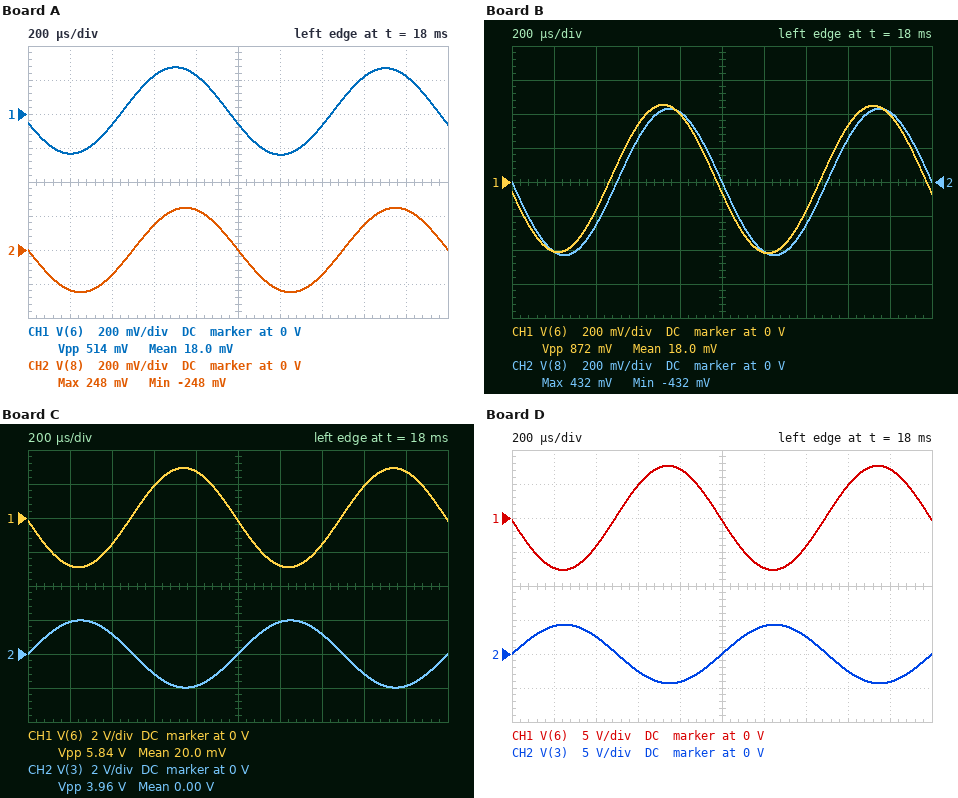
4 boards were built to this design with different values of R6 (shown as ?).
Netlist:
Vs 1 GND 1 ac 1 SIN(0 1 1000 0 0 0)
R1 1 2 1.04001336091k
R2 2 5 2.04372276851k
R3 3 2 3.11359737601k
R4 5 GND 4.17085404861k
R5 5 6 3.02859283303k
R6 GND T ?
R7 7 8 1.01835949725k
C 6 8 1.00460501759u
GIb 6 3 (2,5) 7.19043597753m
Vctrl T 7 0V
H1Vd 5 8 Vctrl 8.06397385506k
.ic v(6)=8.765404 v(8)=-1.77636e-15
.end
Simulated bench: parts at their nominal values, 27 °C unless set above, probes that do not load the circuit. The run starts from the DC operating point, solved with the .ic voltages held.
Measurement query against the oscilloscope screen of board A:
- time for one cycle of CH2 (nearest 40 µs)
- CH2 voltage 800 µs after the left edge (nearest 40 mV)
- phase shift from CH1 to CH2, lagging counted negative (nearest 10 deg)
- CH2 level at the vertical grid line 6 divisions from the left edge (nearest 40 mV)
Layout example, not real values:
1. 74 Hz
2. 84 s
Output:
1. 1.00 ms
2. 240 mV
3. -20 deg
4. -240 mV
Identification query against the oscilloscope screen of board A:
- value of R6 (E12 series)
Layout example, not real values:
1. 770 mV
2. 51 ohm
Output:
1. 680 Ω
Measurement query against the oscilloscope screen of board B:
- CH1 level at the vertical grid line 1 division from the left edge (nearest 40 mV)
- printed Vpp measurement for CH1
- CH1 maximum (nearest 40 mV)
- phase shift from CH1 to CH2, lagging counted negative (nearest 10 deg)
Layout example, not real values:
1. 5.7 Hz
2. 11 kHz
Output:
1. -400 mV
2. 872 mV
3. 440 mV
4. -10 deg
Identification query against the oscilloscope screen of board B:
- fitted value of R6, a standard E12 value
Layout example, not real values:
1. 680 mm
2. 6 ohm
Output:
1. 1.5 kΩ
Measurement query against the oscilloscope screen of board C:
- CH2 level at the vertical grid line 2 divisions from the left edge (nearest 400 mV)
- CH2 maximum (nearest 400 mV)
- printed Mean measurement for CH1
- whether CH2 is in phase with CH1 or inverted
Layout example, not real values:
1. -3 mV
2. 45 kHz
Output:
1. 1.2 V
2. 2.0 V
3. 20.0 mV
4. inverted
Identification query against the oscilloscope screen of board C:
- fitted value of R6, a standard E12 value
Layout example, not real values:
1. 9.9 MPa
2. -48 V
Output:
1. 4.7 kΩ
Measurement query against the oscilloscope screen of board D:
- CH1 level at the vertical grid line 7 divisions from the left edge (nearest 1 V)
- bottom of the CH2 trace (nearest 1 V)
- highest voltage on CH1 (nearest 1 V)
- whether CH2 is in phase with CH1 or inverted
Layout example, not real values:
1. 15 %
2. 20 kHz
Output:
1. -4 V
2. -4 V
3. 8 V
4. inverted
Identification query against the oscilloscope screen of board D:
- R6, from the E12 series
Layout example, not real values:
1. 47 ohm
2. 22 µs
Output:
1. 5.6 kΩ
